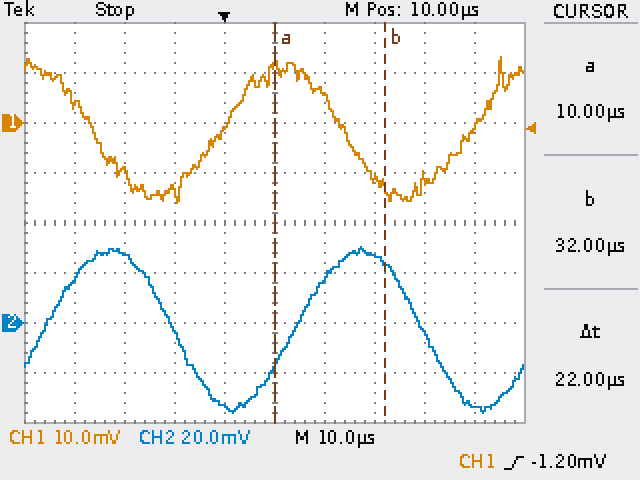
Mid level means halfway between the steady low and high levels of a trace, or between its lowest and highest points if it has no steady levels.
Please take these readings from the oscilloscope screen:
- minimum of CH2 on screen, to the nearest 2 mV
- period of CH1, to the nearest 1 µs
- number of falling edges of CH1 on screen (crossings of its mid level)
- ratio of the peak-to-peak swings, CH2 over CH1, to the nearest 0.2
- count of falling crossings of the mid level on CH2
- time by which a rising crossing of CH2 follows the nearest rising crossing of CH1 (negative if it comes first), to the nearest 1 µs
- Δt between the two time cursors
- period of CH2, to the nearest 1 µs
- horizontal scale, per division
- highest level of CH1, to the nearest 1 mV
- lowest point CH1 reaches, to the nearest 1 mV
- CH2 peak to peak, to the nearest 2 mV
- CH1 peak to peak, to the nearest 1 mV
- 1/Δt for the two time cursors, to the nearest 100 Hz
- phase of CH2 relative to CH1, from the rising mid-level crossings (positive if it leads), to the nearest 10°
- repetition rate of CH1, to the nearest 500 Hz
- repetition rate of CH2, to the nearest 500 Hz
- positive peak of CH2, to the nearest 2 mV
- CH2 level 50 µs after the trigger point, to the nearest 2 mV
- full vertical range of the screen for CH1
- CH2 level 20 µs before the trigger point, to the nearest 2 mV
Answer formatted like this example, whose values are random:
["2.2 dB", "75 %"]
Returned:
["-36 mV", "50 µs", "2", "2.2", "2", "+14 µs", "22 µs", "50 µs", "10 µs", "13 mV", "-16 mV", "66 mV", "29 mV", "45.5 kHz", "-100°", "20.0 kHz", "20.0 kHz", "30 mV", "-34 mV", "80 mV", "28 mV"]
